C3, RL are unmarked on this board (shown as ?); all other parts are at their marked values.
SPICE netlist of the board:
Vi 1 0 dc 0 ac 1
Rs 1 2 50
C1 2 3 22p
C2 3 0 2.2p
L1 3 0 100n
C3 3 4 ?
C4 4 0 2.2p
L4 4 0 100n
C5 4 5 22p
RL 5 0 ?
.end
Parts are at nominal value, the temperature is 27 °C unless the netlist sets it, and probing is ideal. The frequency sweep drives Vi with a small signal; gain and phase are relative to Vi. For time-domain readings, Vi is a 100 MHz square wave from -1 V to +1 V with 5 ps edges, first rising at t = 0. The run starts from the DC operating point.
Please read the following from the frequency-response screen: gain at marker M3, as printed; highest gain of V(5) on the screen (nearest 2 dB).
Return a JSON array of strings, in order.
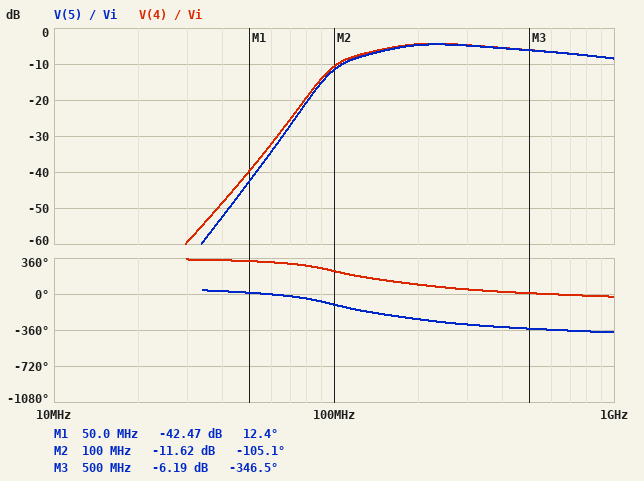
["-6.19 dB", "-4 dB"]
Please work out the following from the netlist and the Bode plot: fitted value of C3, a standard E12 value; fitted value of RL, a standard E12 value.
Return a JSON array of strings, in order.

["3.3 pF", "150 Ω"]
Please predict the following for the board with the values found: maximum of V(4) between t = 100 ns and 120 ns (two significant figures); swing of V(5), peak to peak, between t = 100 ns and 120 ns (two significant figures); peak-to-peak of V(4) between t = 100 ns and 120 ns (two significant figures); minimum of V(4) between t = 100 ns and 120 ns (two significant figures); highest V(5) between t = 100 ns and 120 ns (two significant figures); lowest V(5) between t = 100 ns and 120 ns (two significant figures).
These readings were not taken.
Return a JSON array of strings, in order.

["570 mV", "960 mV", "1.1 V", "-570 mV", "480 mV", "-480 mV"]
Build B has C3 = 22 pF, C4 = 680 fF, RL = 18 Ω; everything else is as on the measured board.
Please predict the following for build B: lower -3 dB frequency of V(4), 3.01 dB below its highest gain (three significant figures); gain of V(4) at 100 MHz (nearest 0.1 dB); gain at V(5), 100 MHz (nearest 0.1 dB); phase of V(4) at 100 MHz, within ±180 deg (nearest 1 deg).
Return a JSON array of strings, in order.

["60.1 MHz", "0.3 dB", "-12.1 dB", "104 deg"]
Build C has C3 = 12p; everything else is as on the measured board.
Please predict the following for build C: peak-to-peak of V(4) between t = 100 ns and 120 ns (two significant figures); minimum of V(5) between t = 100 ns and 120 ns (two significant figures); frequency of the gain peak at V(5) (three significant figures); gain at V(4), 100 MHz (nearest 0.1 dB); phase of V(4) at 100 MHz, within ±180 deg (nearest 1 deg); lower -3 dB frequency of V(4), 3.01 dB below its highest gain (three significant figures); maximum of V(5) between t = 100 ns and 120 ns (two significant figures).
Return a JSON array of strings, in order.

["2.3 V", "-1.2 V", "162 MHz", "-1.6 dB", "154 deg", "75.0 MHz", "1.2 V"]
